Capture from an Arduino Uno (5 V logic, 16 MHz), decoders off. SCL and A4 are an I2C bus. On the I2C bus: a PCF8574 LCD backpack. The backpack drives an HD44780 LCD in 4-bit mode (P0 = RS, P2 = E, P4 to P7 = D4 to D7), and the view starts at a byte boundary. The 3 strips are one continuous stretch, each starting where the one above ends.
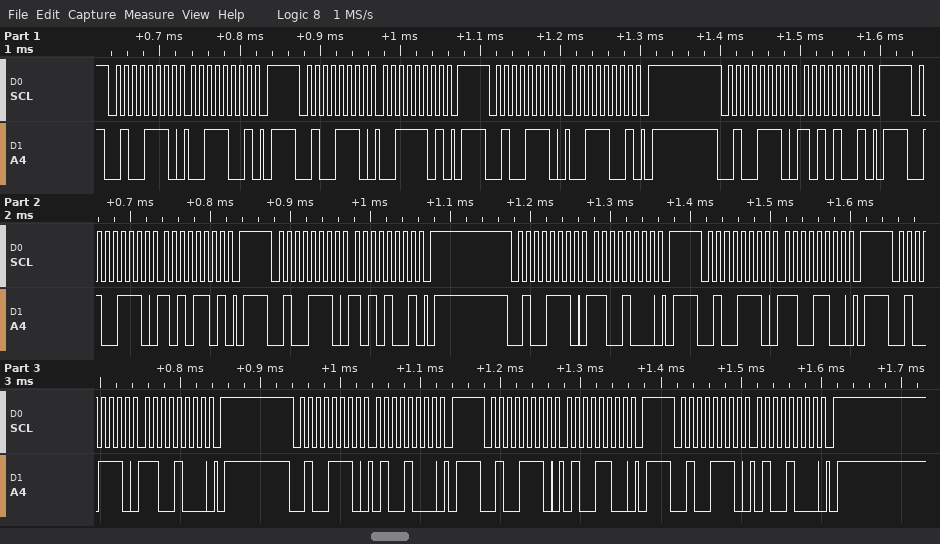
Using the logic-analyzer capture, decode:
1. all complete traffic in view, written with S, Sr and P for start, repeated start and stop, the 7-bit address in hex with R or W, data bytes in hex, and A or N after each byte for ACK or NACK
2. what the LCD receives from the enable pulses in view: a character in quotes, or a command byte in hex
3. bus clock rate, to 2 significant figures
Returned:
S 27W A 39 A P S 27W A 3D A P S 27W A 39 A P S 27W A A9 A P S 27W A AD A P S 27W A A9 A P S 27W A C8 A P S 27W A CC A P S 27W A C8 A P S 27W A 48 A P S 27W A 4C A P S 27W A 48 A P
':' 0xC4
100 kHz
